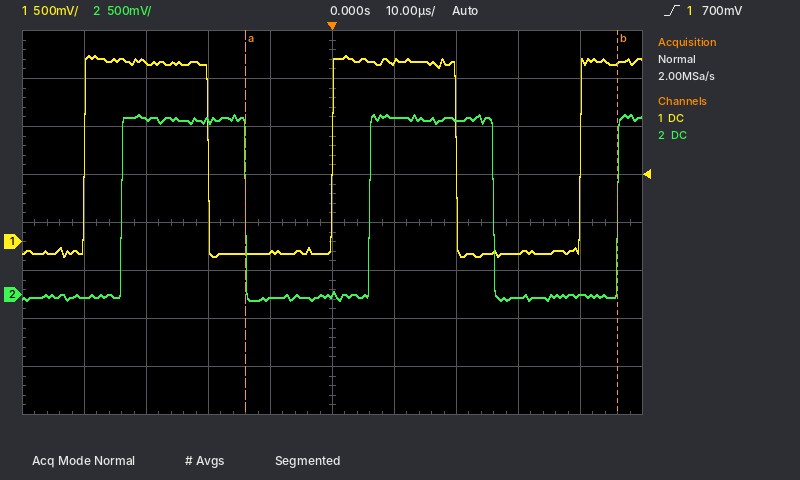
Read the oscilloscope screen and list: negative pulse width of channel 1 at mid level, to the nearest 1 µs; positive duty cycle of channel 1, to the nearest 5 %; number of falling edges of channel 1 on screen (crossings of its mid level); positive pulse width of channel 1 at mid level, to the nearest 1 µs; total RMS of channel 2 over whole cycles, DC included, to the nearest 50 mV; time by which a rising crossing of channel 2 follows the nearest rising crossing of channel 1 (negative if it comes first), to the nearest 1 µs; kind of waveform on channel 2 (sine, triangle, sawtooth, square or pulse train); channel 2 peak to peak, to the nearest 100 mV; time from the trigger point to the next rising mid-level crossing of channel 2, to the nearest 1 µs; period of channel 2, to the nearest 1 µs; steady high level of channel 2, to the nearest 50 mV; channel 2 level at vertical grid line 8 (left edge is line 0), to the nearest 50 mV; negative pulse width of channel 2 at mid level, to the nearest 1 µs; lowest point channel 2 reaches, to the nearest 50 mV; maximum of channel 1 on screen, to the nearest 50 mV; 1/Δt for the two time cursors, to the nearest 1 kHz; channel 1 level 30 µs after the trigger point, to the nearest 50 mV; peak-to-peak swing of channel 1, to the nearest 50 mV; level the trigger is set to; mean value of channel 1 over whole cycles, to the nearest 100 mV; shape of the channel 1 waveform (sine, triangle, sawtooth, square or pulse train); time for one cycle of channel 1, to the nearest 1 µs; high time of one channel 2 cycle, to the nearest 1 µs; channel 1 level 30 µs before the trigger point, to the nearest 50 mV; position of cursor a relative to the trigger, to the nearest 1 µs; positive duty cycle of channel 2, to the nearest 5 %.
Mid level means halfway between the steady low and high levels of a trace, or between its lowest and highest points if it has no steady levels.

20 µs
50 %
2
20 µs
1.30 V
+6 µs
square
1.90 V
6 µs
40 µs
1.85 V
-50 mV
20 µs
-50 mV
1.95 V
17 kHz
-100 mV
2.10 V
700 mV
900 mV
square
40 µs
20 µs
1.85 V
-14 µs
50 %
